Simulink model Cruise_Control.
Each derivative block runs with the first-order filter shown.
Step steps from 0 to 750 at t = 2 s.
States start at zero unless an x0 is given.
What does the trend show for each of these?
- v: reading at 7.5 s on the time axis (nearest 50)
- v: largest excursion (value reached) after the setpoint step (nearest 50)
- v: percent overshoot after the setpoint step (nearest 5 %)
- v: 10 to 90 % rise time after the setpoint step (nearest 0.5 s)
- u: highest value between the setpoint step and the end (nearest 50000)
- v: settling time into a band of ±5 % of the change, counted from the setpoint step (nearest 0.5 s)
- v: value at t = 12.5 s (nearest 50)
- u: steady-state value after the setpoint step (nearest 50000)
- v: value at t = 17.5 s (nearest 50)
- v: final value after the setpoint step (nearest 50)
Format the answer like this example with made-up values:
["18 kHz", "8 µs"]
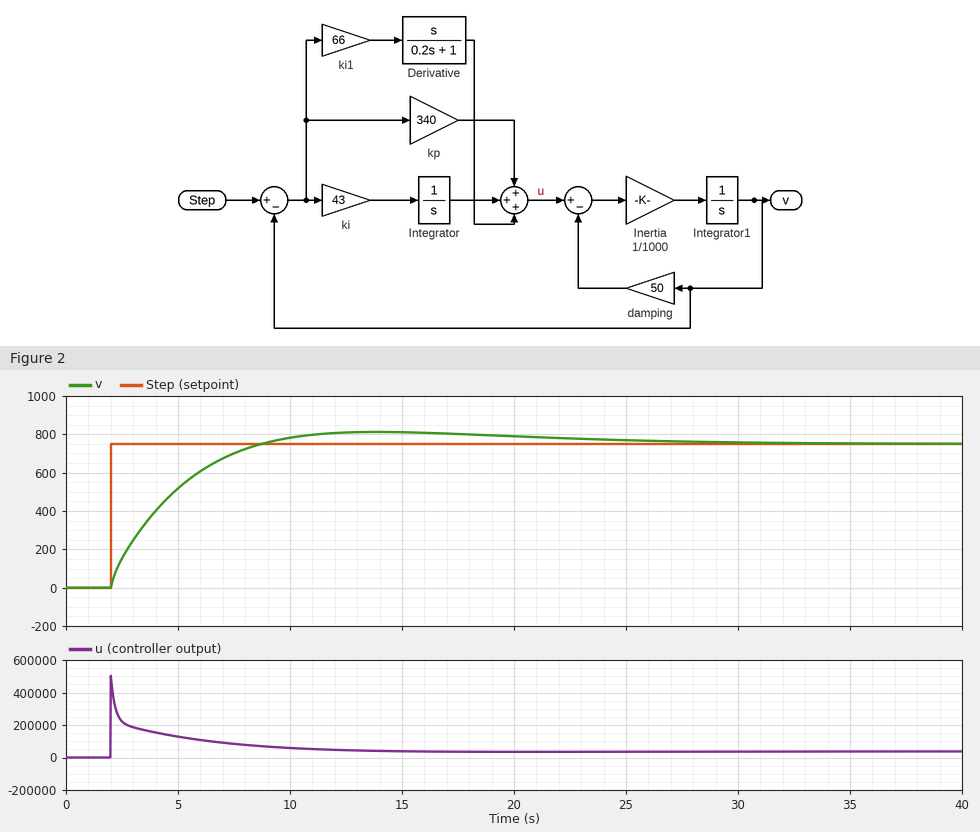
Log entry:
["700", "800", "10 %", "5.0 s", "500000", "18.5 s", "800", "50000", "800", "750"]
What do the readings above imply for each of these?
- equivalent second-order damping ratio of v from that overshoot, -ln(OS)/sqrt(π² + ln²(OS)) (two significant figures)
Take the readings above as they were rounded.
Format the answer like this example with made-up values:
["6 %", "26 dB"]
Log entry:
["0.59"]
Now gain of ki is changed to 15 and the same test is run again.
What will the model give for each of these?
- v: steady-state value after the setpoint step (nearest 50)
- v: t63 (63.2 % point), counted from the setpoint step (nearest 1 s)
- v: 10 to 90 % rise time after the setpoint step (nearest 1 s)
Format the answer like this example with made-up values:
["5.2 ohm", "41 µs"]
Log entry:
["750", "3 s", "7 s"]
